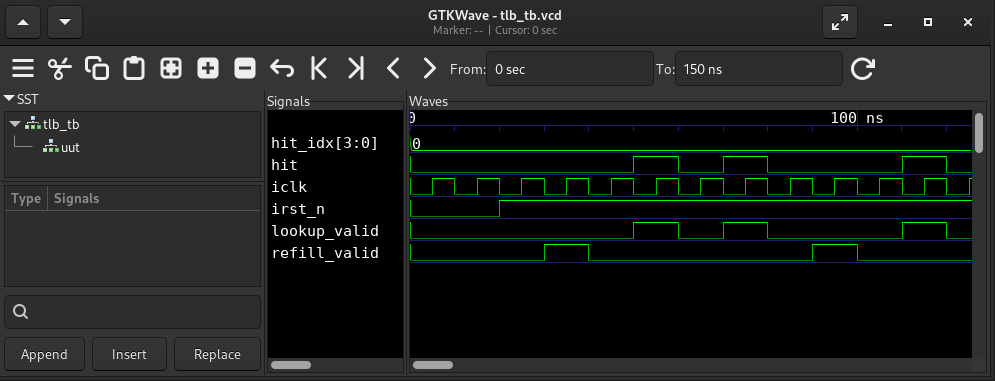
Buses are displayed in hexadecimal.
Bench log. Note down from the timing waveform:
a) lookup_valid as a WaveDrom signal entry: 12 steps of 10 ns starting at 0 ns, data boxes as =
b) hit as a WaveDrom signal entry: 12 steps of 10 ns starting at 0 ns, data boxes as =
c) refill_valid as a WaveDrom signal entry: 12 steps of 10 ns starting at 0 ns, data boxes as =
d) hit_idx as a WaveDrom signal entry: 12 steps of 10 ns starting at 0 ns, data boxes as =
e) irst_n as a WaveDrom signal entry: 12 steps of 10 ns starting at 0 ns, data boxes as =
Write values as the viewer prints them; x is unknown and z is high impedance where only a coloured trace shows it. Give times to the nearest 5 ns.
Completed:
{name: 'lookup_valid', wave: '0....1010..1'}
{name: 'hit', wave: '0....1010..1'}
{name: 'refill_valid', wave: '0..10....10.'}
{name: 'hit_idx', wave: '=...........', data: '0'}
{name: 'irst_n', wave: '0.1.........'}
